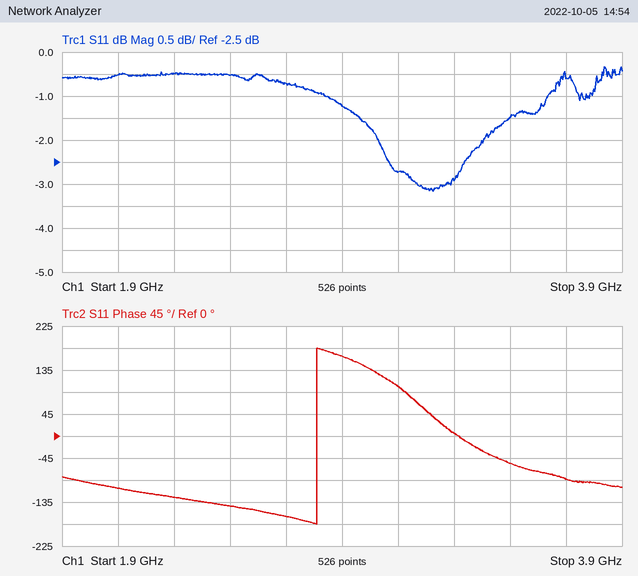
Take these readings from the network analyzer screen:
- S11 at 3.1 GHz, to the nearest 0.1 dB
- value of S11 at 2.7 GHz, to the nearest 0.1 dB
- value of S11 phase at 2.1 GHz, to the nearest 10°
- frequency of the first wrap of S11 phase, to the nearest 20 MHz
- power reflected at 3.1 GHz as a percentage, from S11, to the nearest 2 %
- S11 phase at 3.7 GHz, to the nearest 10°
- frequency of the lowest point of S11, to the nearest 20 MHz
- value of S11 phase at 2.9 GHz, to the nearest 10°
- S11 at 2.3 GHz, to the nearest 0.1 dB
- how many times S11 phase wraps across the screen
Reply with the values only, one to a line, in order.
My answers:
-2.7 dB
-0.7 dB
-110°
2.80 GHz
54 %
-90°
3.22 GHz
160°
-0.5 dB
1
